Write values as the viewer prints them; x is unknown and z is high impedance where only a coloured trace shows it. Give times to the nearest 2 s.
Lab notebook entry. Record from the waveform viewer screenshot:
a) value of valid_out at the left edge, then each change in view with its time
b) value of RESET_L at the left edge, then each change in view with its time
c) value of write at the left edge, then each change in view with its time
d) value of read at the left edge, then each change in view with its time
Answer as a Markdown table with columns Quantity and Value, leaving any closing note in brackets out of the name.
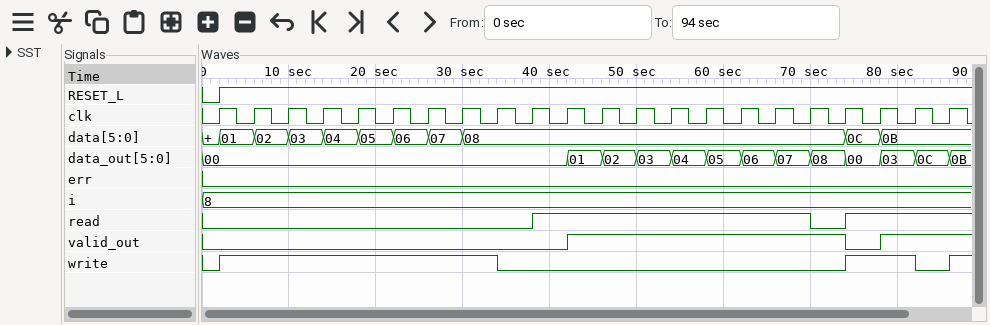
| Quantity | Value |
|---|---|
| value of valid_out at the left edge, then each change in view with its time | 0, 1 at 42 s, 0 at 74 s, 1 at 78 s |
| value of RESET_L at the left edge, then each change in view with its time | 0, 1 at 2 s |
| value of write at the left edge, then each change in view with its time | 0, 1 at 2 s, 0 at 34 s, 1 at 74 s, 0 at 82 s, 1 at 86 s |
| value of read at the left edge, then each change in view with its time | 0, 1 at 38 s, 0 at 70 s, 1 at 74 s |
